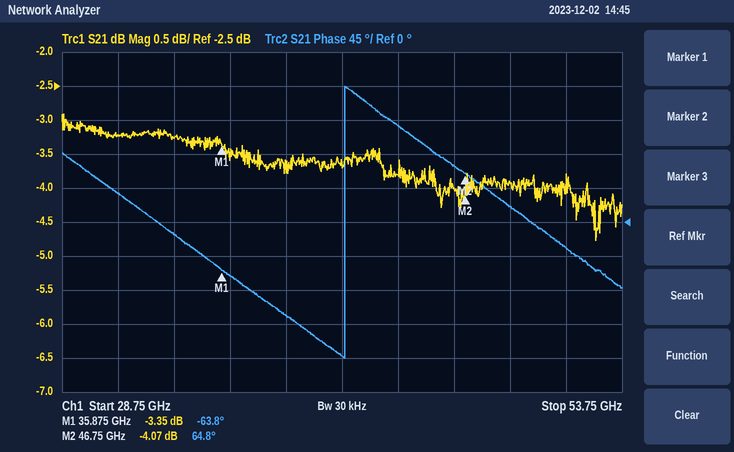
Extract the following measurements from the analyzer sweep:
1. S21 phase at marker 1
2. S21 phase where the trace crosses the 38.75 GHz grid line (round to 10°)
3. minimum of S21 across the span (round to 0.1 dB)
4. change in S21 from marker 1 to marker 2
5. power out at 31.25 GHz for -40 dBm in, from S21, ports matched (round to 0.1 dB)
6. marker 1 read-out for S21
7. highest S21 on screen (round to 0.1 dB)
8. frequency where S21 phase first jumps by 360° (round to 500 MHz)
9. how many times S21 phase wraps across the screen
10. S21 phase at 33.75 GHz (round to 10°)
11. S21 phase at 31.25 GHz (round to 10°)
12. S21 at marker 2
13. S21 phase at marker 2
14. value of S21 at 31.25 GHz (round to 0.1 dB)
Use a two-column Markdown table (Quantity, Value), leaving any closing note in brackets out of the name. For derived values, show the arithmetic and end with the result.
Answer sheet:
| Quantity | Value |
|---|---|
| S21 phase at marker 1 | -63.8° |
| S21 phase where the trace crosses the 38.75 GHz grid line | -120° |
| minimum of S21 across the span | -4.8 dB |
| change in S21 from marker 1 to marker 2 | -4.07 − (-3.35) = -0.72 dB |
| power out at 31.25 GHz for -40 dBm in, from S21, ports matched | -40 dBm + (-3.2 dB) = -43.2 dBm |
| marker 1 read-out for S21 | -3.35 dB |
| highest S21 on screen | -2.9 dB |
| frequency where S21 phase first jumps by 360° | 41.5 GHz |
| how many times S21 phase wraps across the screen | 1 |
| S21 phase at 33.75 GHz | -20° |
| S21 phase at 31.25 GHz | 40° |
| S21 at marker 2 | -4.07 dB |
| S21 phase at marker 2 | 64.8° |
| value of S21 at 31.25 GHz | -3.2 dB |
